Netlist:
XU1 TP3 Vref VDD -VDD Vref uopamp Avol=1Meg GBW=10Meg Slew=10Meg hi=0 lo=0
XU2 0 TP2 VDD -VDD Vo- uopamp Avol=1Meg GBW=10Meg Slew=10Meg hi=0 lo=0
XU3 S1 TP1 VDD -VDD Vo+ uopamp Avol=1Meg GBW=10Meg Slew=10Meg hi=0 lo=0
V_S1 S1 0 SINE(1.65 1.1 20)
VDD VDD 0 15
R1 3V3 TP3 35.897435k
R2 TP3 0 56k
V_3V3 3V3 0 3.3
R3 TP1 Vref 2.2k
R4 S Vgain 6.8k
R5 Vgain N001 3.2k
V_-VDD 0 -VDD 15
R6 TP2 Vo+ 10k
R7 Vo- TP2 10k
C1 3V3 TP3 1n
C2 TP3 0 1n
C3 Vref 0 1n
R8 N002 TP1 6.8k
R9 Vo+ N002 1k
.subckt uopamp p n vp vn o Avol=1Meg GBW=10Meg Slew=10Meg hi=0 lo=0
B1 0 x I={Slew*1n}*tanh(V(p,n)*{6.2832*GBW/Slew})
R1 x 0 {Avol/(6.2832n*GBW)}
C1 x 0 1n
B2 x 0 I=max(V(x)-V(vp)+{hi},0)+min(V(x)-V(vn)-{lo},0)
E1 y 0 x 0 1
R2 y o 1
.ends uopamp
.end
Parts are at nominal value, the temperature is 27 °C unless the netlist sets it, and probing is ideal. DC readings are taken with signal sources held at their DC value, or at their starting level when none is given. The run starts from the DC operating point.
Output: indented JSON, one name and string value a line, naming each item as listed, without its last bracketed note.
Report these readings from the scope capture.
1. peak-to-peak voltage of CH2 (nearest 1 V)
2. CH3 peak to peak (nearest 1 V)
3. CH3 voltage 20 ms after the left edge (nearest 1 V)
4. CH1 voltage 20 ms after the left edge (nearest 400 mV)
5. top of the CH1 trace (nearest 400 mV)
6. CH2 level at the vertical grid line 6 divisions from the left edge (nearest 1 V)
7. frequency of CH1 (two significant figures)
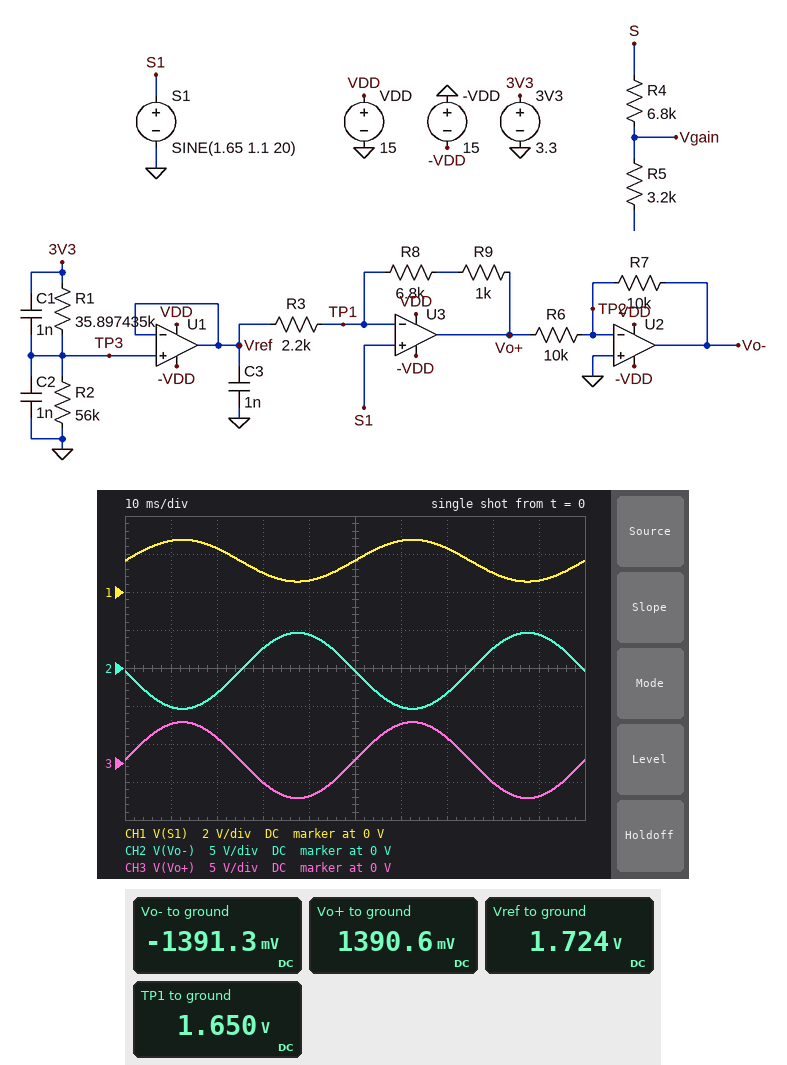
{
  "peak-to-peak voltage of CH2": "10 V",
  "CH3 peak to peak": "10 V",
  "CH3 voltage 20 ms after the left edge": "3 V",
  "CH1 voltage 20 ms after the left edge": "2.4 V",
  "top of the CH1 trace": "2.8 V",
  "CH2 level at the vertical grid line 6 divisions from the left edge": "-5 V",
  "frequency of CH1": "20 Hz"
}
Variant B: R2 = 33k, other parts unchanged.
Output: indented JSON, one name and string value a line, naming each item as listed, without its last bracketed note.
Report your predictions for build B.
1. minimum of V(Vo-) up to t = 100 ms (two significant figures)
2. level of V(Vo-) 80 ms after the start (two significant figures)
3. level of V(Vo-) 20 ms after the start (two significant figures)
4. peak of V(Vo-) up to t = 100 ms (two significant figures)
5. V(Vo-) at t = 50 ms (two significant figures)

{
  "minimum of V(Vo-) up to t = 100 ms": "-6.9 V",
  "level of V(Vo-) 80 ms after the start": "1.0 V",
  "level of V(Vo-) 20 ms after the start": "-4.8 V",
  "peak of V(Vo-) up to t = 100 ms": "3.1 V",
  "V(Vo-) at t = 50 ms": "-1.9 V"
}
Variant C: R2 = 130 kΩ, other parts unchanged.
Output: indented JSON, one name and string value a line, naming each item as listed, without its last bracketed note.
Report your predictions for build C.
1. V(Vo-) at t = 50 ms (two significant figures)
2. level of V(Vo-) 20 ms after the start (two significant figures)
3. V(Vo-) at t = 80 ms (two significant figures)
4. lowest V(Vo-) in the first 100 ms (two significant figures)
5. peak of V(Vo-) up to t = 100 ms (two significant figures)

{
  "V(Vo-) at t = 50 ms": "1.7 V",
  "level of V(Vo-) 20 ms after the start": "-1.3 V",
  "V(Vo-) at t = 80 ms": "4.6 V",
  "lowest V(Vo-) in the first 100 ms": "-3.3 V",
  "peak of V(Vo-) up to t = 100 ms": "6.7 V"
}
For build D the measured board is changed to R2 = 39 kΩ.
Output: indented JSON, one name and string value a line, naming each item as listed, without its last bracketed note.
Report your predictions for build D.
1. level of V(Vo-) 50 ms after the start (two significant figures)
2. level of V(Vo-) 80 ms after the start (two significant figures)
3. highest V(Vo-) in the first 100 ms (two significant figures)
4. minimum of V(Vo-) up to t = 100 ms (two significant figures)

{
  "level of V(Vo-) 50 ms after the start": "-1.4 V",
  "level of V(Vo-) 80 ms after the start": "1.5 V",
  "highest V(Vo-) in the first 100 ms": "3.6 V",
  "minimum of V(Vo-) up to t = 100 ms": "-6.4 V"
}
